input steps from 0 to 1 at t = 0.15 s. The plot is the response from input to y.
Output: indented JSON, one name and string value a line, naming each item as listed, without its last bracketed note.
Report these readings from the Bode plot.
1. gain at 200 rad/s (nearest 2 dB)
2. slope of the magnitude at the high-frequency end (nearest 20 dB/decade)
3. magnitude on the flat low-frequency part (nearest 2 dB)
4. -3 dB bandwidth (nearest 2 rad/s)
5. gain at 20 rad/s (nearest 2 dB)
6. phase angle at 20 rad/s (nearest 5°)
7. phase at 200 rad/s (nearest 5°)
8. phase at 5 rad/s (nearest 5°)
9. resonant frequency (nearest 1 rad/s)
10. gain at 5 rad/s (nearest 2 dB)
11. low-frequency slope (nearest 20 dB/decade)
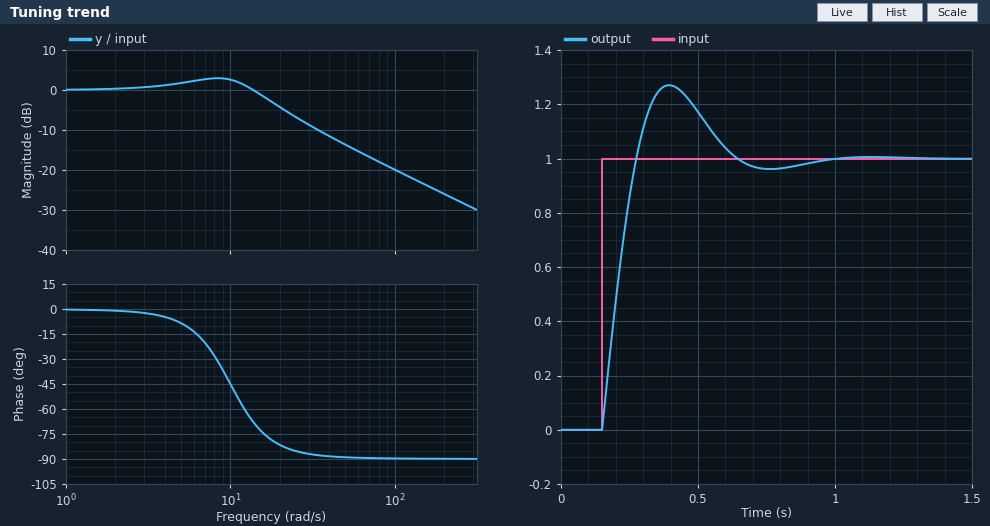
{
  "gain at 200 rad/s": "-26 dB",
  "slope of the magnitude at the high-frequency end": "-20 dB/decade",
  "magnitude on the flat low-frequency part": "0 dB",
  "-3 dB bandwidth": "18 rad/s",
  "gain at 20 rad/s": "-4 dB",
  "phase angle at 20 rad/s": "-80°",
  "phase at 200 rad/s": "-90°",
  "phase at 5 rad/s": "-10°",
  "resonant frequency": "8 rad/s",
  "gain at 5 rad/s": "2 dB",
  "low-frequency slope": "0 dB/decade"
}
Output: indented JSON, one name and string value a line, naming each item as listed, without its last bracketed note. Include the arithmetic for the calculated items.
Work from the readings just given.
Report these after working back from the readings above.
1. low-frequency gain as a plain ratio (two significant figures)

{
  "low-frequency gain as a plain ratio": "10^(0 / 20) = 1.0"
}
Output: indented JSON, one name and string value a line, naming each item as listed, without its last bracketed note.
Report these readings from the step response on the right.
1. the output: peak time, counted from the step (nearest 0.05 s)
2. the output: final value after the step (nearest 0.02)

{
  "the output: peak time, counted from the step": "0.25 s",
  "the output: final value after the step": "1.00"
}
